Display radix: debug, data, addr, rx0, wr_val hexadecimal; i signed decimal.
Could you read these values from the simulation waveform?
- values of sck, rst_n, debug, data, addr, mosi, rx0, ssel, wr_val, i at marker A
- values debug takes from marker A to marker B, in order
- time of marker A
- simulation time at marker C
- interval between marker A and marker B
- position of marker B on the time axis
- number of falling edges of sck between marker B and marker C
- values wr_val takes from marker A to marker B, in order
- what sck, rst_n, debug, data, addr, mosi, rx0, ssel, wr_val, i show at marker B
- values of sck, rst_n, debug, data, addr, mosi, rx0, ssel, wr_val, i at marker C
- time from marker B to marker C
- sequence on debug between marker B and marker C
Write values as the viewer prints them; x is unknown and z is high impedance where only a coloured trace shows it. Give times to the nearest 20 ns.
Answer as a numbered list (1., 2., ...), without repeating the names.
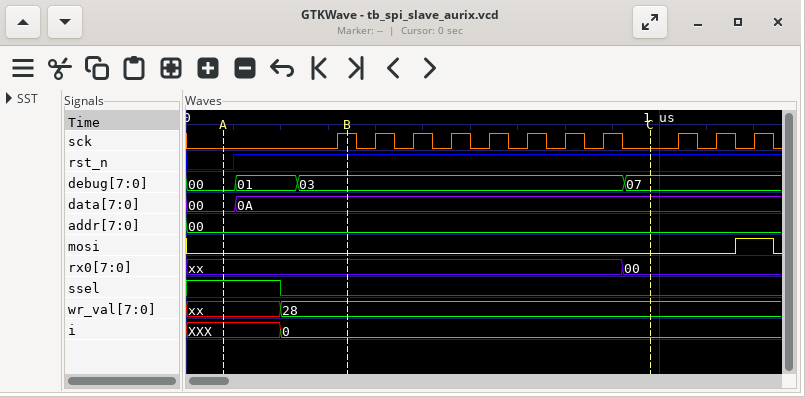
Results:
1. sck=0, rst_n=0, debug=00, data=00, addr=00, mosi=0, rx0=xx, ssel=1, wr_val=xx, i=XXX
2. 00, 01, 03
3. 80 ns
4. 980 ns
5. 260 ns
6. 340 ns
7. 8
8. xx, 28
9. sck=1, rst_n=1, debug=03, data=0A, addr=00, mosi=0, rx0=xx, ssel=0, wr_val=28, i=0
10. sck=0, rst_n=1, debug=07, data=0A, addr=00, mosi=0, rx0=00, ssel=0, wr_val=28, i=0
11. 640 ns
12. 03, 07
